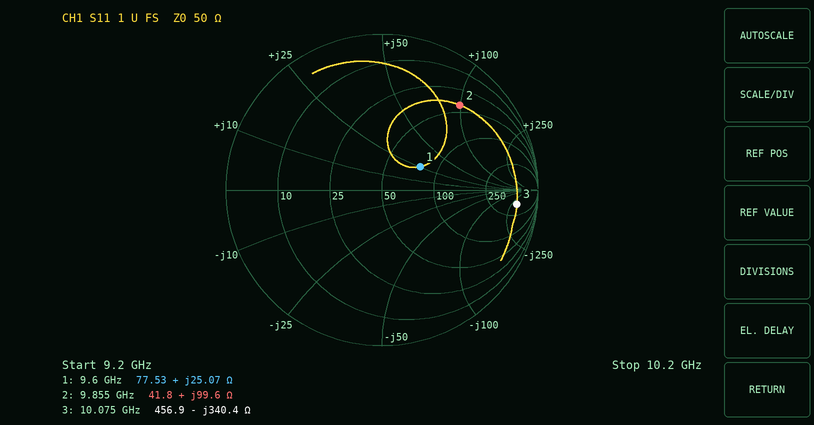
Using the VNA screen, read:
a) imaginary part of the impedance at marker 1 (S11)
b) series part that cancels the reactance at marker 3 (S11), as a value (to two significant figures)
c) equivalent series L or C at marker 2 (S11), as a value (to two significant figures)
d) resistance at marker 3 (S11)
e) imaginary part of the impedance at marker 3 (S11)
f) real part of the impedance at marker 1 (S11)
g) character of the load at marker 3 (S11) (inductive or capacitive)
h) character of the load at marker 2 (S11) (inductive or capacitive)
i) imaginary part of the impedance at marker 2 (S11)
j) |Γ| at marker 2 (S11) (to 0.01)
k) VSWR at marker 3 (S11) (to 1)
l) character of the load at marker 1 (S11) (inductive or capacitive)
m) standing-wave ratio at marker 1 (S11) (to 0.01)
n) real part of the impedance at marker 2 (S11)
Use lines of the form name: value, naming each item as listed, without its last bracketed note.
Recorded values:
imaginary part of the impedance at marker 1: +25.07 Ω
series part that cancels the reactance at marker 3 (S11), as a value: 5.4 nH
equivalent series L or C at marker 2 (S11), as a value: 1.6 nH
resistance at marker 3: 456.9 Ω
imaginary part of the impedance at marker 3: -340.4 Ω
real part of the impedance at marker 1: 77.53 Ω
character of the load at marker 3 (S11): capacitive
character of the load at marker 2 (S11): inductive
imaginary part of the impedance at marker 2: +99.6 Ω
|Γ| at marker 2 (S11): 0.74
VSWR at marker 3 (S11): 14
character of the load at marker 1 (S11): inductive
standing-wave ratio at marker 1 (S11): 1.80
real part of the impedance at marker 2: 41.8 Ω
